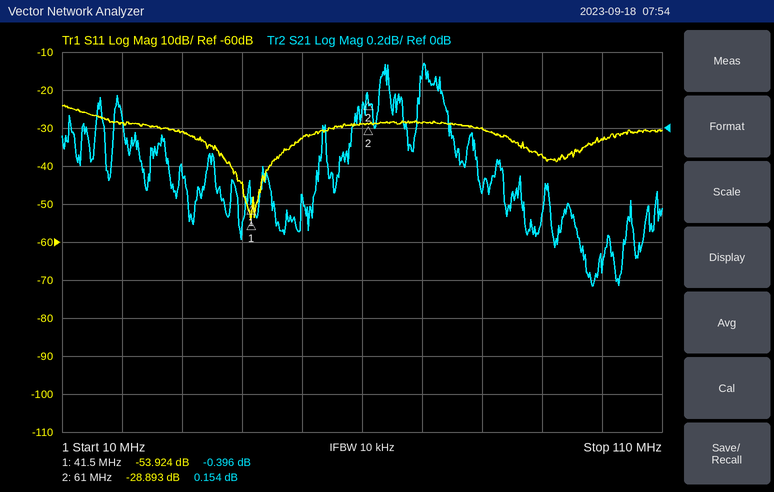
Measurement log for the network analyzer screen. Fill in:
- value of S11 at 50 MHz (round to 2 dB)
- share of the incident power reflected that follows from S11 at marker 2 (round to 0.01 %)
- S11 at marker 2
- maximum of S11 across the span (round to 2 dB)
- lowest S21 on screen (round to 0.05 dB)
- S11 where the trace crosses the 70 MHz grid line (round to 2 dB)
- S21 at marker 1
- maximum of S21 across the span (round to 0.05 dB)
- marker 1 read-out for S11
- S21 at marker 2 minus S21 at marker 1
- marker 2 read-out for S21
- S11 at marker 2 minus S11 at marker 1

-32 dB
0.13 %
-28.893 dB
-24 dB
-0.85 dB
-28 dB
-0.396 dB
0.35 dB
-53.924 dB
0.550 dB
0.154 dB
25.031 dB
